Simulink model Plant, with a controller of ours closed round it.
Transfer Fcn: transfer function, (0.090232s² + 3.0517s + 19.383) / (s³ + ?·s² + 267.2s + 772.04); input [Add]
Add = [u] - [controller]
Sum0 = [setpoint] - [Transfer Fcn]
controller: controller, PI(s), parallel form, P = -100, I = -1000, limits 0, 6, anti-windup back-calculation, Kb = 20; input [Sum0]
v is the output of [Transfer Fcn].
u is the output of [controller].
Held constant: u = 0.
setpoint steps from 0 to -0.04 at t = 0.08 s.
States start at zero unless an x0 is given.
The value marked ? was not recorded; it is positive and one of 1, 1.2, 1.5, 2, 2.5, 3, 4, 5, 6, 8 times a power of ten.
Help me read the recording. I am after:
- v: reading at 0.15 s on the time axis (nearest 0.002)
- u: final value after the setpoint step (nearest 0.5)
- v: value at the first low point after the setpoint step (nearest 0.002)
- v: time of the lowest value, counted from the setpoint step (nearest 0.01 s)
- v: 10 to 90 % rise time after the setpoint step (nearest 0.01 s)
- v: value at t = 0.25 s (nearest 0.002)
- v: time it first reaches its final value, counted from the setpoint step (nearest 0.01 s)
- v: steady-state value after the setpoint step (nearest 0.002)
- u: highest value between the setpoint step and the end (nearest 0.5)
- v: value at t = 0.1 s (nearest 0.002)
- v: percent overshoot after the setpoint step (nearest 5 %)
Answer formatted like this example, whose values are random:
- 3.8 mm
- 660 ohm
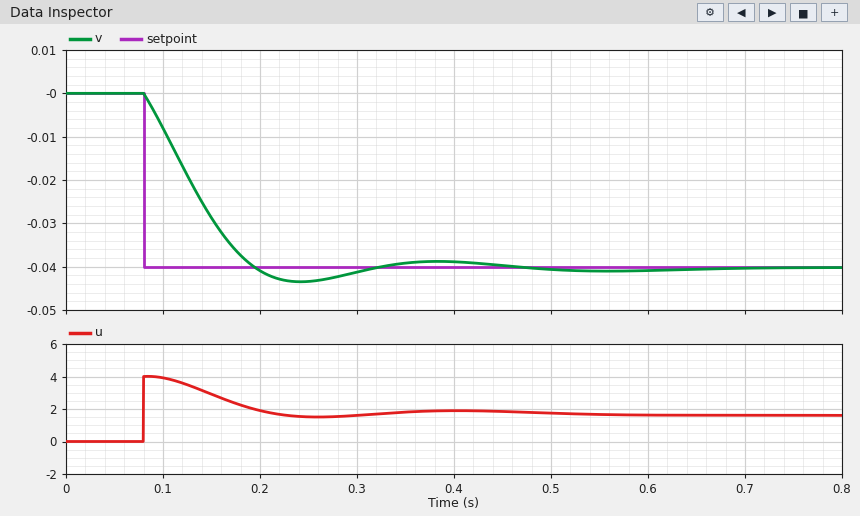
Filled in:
- -0.028
- 1.5
- -0.044
- 0.16 s
- 0.08 s
- -0.044
- 0.11 s
- -0.040
- 4.0
- -0.008
- 10 %
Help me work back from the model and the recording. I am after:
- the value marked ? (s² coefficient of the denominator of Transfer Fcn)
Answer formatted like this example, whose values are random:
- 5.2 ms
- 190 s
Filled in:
- 20
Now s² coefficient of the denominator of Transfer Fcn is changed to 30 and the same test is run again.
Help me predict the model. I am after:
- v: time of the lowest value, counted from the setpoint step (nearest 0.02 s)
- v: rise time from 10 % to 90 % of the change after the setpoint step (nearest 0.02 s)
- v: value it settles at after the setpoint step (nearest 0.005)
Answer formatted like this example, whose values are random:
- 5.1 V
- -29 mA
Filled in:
- 0.22 s
- 0.10 s
- -0.040
